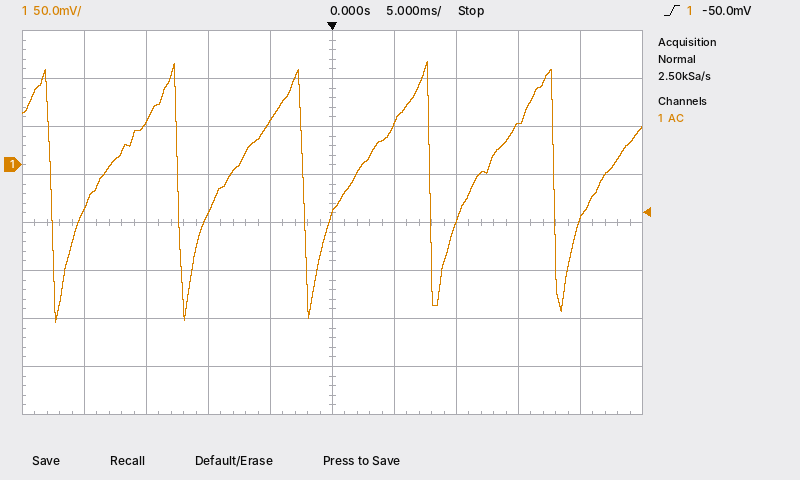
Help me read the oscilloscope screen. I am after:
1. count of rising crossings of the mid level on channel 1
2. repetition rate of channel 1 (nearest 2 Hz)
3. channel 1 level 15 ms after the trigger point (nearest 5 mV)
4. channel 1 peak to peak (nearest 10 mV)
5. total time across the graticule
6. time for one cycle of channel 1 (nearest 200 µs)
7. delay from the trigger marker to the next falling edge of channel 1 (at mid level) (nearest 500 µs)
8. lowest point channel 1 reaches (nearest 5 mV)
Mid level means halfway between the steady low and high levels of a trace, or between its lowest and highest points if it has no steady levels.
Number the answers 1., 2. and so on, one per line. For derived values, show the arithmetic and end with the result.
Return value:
1. 5
2. 1 / 10.2 ms ≈ 98 Hz
3. 40 mV
4. 270 mV
5. 50 ms
6. 10.2 ms
7. 8.0 ms
8. -165 mV
